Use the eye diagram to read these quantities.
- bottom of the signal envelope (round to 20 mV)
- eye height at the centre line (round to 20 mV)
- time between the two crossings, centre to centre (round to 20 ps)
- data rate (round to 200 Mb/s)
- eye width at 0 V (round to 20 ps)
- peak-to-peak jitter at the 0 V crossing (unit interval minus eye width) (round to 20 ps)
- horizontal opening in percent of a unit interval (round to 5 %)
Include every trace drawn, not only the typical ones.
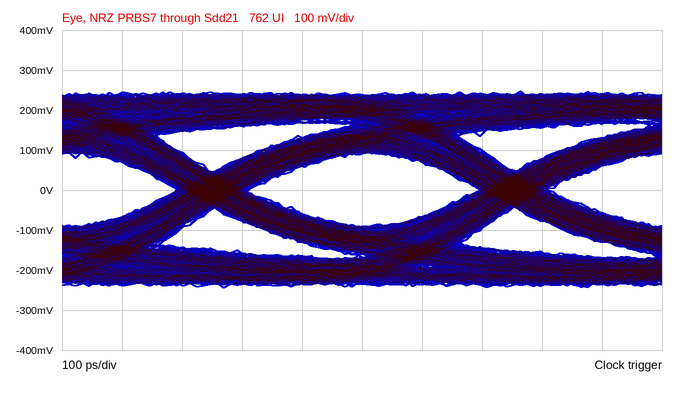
-240 mV
180 mV
500 ps
2.0 Gb/s
380 ps
120 ps
75 %
